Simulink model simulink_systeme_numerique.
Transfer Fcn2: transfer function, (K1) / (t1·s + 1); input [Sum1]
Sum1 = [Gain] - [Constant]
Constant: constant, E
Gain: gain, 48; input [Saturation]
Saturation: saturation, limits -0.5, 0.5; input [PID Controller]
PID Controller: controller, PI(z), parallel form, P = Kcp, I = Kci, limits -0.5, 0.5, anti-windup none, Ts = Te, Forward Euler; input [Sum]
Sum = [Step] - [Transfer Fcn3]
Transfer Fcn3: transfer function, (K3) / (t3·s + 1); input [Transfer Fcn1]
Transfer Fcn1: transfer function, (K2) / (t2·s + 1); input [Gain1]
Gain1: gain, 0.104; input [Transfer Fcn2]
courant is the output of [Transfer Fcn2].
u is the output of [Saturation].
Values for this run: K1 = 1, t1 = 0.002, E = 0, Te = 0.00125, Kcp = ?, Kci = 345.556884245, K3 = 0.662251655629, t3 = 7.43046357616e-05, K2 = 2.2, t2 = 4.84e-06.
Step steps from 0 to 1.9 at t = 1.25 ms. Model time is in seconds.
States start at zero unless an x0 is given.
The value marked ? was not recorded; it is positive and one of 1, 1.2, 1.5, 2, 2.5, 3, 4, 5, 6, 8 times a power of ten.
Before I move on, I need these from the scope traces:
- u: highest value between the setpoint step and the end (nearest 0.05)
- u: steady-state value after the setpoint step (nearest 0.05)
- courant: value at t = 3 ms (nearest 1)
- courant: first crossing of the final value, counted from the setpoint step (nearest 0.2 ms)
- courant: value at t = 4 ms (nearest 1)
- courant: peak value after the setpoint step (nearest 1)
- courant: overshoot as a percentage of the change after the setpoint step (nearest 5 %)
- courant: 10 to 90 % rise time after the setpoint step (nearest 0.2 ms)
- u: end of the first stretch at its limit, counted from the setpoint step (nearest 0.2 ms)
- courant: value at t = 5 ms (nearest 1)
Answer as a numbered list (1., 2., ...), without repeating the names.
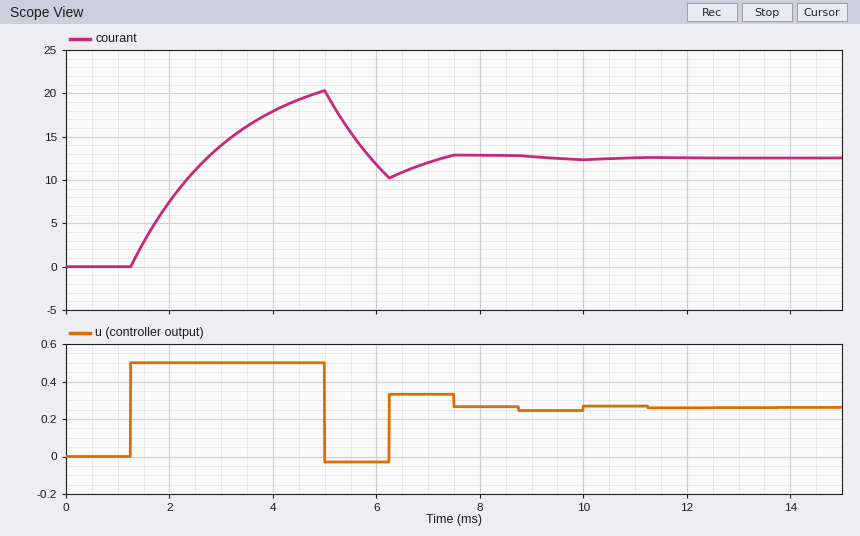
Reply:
1. 0.50
2. 0.25
3. 14
4. 1.4 ms
5. 18
6. 20
7. 60 %
8. 1.2 ms
9. 3.8 ms
10. 20
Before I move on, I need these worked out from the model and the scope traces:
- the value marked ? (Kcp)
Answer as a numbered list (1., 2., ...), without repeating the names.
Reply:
1. 0.6
